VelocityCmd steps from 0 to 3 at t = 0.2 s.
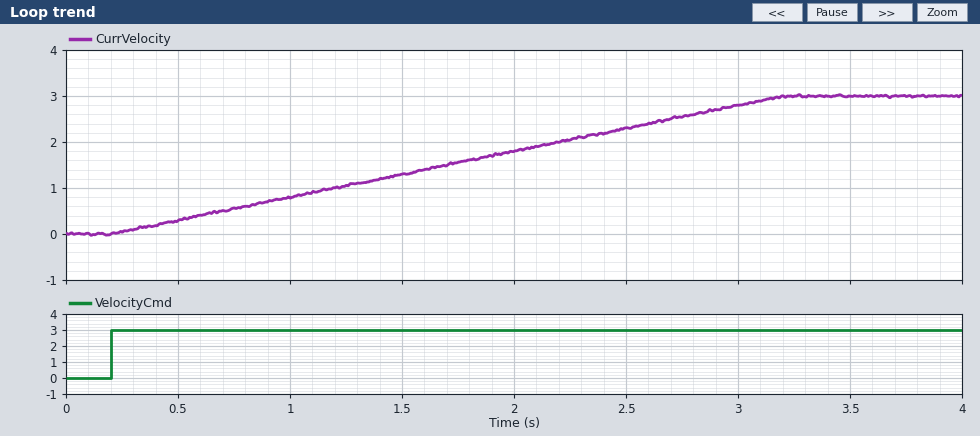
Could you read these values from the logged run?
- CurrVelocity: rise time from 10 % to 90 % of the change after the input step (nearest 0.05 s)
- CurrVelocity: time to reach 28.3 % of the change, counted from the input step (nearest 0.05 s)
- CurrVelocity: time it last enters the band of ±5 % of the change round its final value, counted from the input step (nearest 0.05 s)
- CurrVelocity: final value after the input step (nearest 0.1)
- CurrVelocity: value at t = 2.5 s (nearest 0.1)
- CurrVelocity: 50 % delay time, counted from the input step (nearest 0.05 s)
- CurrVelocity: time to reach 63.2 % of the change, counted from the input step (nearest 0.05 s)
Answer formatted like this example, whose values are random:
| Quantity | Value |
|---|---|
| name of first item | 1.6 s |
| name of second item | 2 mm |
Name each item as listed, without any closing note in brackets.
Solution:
| Quantity | Value |
|---|---|
| CurrVelocity: rise time from 10 % to 90 % of the change after the input step | 2.40 s |
| CurrVelocity: time to reach 28.3 % of the change, counted from the input step | 0.85 s |
| CurrVelocity: time it last enters the band of ±5 % of the change round its final value, counted from the input step | 2.85 s |
| CurrVelocity: final value after the input step | 3.0 |
| CurrVelocity: value at t = 2.5 s | 2.3 |
| CurrVelocity: 50 % delay time, counted from the input step | 1.50 s |
| CurrVelocity: time to reach 63.2 % of the change, counted from the input step | 1.90 s |
